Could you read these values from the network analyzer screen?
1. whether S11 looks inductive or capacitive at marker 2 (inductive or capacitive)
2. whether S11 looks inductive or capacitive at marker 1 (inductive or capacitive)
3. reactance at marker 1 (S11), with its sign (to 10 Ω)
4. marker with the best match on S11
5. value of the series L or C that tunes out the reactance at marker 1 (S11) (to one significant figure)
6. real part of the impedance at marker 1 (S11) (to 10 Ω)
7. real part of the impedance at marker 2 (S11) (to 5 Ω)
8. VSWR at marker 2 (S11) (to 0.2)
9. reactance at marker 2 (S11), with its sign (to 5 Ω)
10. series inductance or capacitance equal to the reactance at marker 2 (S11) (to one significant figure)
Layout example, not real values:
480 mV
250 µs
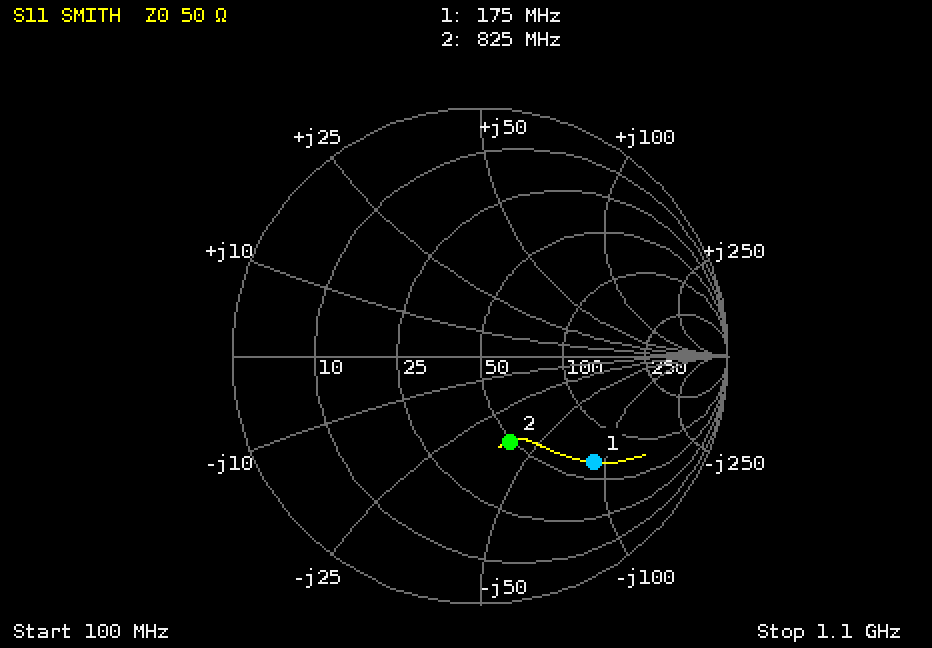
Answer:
capacitive
capacitive
-90 Ω
marker 2
80 nH
60 Ω
50 Ω
2.2
-40 Ω
5 pF
